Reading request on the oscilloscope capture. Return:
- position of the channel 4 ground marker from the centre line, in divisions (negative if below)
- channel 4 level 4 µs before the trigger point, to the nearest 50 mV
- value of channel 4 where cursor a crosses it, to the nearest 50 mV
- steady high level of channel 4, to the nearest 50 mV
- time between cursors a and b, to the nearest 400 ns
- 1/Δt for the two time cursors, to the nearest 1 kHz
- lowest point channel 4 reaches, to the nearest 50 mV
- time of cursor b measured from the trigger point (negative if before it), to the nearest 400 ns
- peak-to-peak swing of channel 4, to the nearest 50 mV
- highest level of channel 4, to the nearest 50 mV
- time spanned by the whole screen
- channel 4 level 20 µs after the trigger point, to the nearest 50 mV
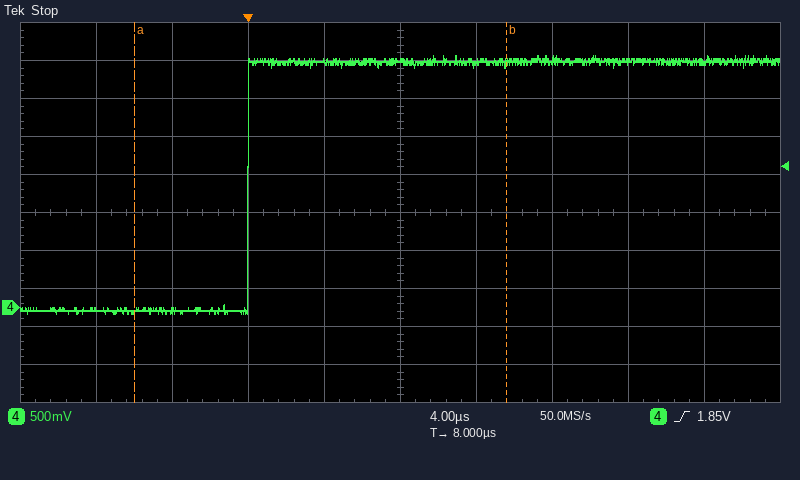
-2.5 div
-50 mV
-50 mV
3.25 V
19.6 µs
51 kHz
-100 mV
+13.6 µs
3.40 V
3.30 V
40 µs
3.25 V
